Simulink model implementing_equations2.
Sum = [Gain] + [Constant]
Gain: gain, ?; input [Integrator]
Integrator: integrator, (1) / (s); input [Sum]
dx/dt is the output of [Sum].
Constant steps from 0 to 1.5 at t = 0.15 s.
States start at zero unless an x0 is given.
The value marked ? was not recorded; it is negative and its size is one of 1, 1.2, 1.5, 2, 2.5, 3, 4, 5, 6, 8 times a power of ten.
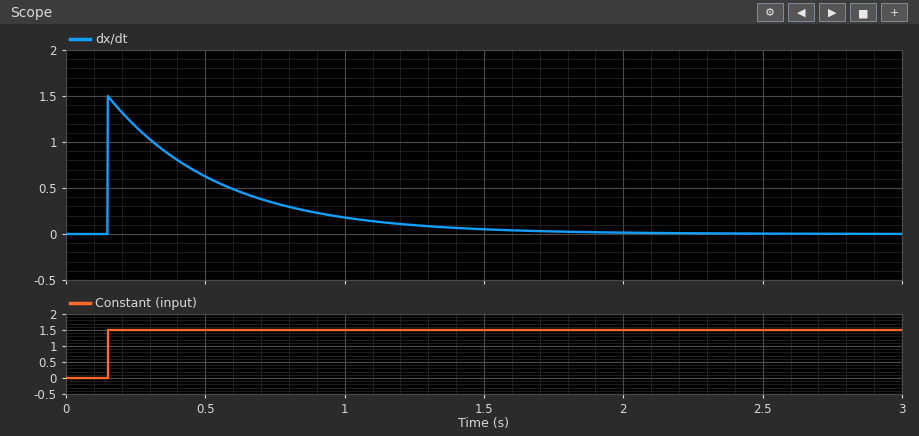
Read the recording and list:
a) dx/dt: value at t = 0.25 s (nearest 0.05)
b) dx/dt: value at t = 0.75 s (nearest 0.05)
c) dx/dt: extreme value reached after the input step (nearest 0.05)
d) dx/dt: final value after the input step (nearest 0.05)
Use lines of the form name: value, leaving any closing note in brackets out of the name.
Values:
dx/dt: value at t = 0.25 s: 1.15
dx/dt: value at t = 0.75 s: 0.35
dx/dt: extreme value reached after the input step: 1.50
dx/dt: final value after the input step: 0.00
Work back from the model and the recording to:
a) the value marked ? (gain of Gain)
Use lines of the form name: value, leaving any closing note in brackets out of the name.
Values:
the value marked ?: -2.5
